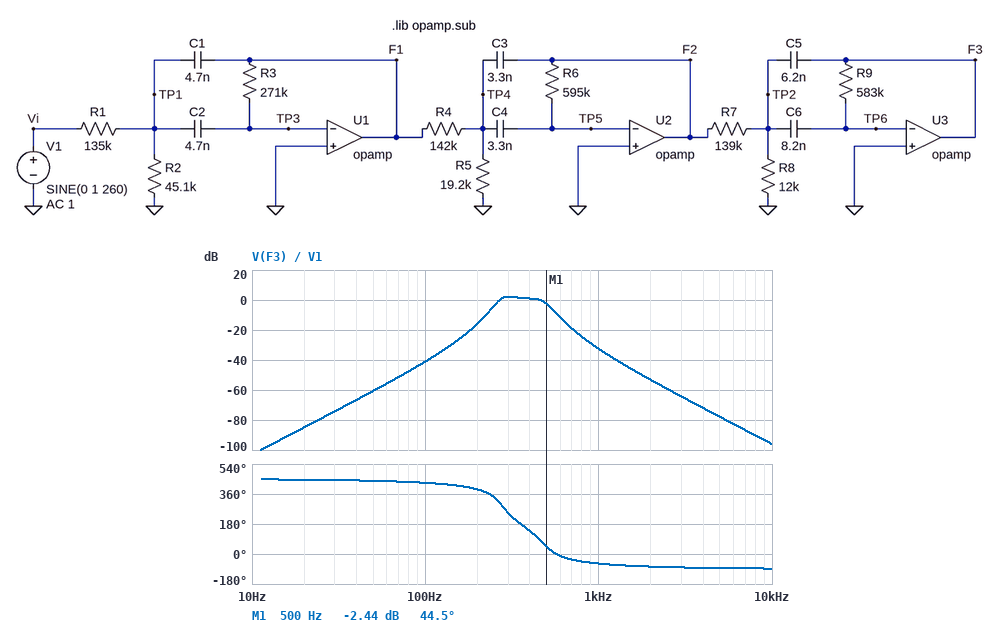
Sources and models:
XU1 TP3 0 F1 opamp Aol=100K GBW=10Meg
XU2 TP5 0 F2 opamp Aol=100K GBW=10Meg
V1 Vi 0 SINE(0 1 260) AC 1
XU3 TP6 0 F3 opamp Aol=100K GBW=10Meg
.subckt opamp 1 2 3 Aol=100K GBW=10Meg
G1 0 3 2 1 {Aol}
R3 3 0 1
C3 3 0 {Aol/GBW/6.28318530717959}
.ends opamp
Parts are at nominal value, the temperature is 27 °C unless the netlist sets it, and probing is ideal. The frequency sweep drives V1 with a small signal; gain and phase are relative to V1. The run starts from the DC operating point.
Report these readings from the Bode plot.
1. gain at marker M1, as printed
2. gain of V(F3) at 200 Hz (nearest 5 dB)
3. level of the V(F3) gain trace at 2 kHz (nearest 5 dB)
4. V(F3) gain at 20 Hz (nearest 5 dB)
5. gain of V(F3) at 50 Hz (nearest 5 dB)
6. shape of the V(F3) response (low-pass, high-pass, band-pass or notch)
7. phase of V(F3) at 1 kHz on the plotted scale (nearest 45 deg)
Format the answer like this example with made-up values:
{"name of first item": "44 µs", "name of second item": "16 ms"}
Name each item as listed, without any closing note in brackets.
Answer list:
{"gain at marker M1, as printed": "-2.44 dB", "gain of V(F3) at 200 Hz": "-15 dB", "level of the V(F3) gain trace at 2 kHz": "-55 dB", "V(F3) gain at 20 Hz": "-85 dB", "gain of V(F3) at 50 Hz": "-60 dB", "shape of the V(F3) response": "band-pass", "phase of V(F3) at 1 kHz on the plotted scale": "-45 deg"}
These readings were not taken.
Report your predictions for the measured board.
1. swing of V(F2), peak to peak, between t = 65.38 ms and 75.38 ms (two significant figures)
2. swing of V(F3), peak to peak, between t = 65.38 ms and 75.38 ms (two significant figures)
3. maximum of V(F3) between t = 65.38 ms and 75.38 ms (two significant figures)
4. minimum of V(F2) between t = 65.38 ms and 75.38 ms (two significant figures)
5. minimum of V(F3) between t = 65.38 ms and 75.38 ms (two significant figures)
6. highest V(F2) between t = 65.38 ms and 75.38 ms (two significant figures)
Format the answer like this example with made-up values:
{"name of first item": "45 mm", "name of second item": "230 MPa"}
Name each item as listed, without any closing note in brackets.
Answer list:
{"swing of V(F2), peak to peak, between t = 65.38 ms and 75.38 ms": "790 mV", "swing of V(F3), peak to peak, between t = 65.38 ms and 75.38 ms": "1.7 V", "maximum of V(F3) between t = 65.38 ms and 75.38 ms": "840 mV", "minimum of V(F2) between t = 65.38 ms and 75.38 ms": "-390 mV", "minimum of V(F3) between t = 65.38 ms and 75.38 ms": "-840 mV", "highest V(F2) between t = 65.38 ms and 75.38 ms": "390 mV"}
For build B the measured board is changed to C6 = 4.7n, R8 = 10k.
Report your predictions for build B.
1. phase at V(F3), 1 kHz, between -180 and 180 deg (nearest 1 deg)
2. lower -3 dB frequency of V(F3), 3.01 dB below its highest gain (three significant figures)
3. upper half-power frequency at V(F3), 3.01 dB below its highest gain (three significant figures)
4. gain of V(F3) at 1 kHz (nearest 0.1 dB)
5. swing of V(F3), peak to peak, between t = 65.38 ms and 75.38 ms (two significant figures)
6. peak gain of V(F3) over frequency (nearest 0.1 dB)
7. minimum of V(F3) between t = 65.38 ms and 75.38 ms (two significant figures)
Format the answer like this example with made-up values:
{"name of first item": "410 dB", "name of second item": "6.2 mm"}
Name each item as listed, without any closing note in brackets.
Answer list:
{"phase at V(F3), 1 kHz, between -180 and 180 deg": "-55 deg", "lower -3 dB frequency of V(F3), 3.01 dB below its highest gain": "371 Hz", "upper half-power frequency at V(F3), 3.01 dB below its highest gain": "472 Hz", "gain of V(F3) at 1 kHz": "-31.7 dB", "swing of V(F3), peak to peak, between t = 65.38 ms and 75.38 ms": "390 mV", "peak gain of V(F3) over frequency": "8.0 dB", "minimum of V(F3) between t = 65.38 ms and 75.38 ms": "-200 mV"}
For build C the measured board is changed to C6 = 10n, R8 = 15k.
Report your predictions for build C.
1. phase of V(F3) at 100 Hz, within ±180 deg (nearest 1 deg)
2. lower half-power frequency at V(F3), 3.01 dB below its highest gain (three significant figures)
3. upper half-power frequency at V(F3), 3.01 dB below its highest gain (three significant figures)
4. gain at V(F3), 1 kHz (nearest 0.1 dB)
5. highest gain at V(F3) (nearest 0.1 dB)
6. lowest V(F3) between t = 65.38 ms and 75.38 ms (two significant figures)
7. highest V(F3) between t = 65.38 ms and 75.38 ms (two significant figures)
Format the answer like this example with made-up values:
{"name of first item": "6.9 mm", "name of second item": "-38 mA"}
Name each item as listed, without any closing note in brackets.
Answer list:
{"phase of V(F3) at 100 Hz, within ±180 deg": "64 deg", "lower half-power frequency at V(F3), 3.01 dB below its highest gain": "223 Hz", "upper half-power frequency at V(F3), 3.01 dB below its highest gain": "506 Hz", "gain at V(F3), 1 kHz": "-32.7 dB", "highest gain at V(F3)": "-1.0 dB", "lowest V(F3) between t = 65.38 ms and 75.38 ms": "-770 mV", "highest V(F3) between t = 65.38 ms and 75.38 ms": "770 mV"}
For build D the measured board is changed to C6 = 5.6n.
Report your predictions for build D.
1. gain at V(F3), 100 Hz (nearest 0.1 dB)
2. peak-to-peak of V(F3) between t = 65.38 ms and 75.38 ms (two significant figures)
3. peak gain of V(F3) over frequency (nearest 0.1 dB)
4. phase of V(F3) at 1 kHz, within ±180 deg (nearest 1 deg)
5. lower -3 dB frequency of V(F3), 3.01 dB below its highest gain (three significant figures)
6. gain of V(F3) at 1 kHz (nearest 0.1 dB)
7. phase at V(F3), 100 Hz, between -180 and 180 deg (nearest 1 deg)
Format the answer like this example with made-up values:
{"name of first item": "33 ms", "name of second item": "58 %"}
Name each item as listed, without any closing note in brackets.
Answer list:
{"gain at V(F3), 100 Hz": "-44.7 dB", "peak-to-peak of V(F3) between t = 65.38 ms and 75.38 ms": "730 mV", "peak gain of V(F3) over frequency": "5.5 dB", "phase of V(F3) at 1 kHz, within ±180 deg": "-56 deg", "lower -3 dB frequency of V(F3), 3.01 dB below its highest gain": "316 Hz", "gain of V(F3) at 1 kHz": "-32.2 dB", "phase at V(F3), 100 Hz, between -180 and 180 deg": "68 deg"}
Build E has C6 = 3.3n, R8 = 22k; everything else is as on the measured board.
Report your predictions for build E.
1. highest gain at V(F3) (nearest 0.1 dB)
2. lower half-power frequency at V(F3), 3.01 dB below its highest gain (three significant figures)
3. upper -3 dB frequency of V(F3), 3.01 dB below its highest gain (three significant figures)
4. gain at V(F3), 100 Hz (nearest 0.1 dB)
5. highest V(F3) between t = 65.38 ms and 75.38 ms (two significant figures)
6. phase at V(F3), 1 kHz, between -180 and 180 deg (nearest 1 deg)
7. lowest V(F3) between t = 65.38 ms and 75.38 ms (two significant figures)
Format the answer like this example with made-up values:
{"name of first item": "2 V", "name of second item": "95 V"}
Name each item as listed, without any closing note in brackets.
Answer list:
{"highest gain at V(F3)": "3.2 dB", "lower half-power frequency at V(F3), 3.01 dB below its highest gain": "316 Hz", "upper -3 dB frequency of V(F3), 3.01 dB below its highest gain": "484 Hz", "gain at V(F3), 100 Hz": "-44.6 dB", "highest V(F3) between t = 65.38 ms and 75.38 ms": "340 mV", "phase at V(F3), 1 kHz, between -180 and 180 deg": "-54 deg", "lowest V(F3) between t = 65.38 ms and 75.38 ms": "-340 mV"}
